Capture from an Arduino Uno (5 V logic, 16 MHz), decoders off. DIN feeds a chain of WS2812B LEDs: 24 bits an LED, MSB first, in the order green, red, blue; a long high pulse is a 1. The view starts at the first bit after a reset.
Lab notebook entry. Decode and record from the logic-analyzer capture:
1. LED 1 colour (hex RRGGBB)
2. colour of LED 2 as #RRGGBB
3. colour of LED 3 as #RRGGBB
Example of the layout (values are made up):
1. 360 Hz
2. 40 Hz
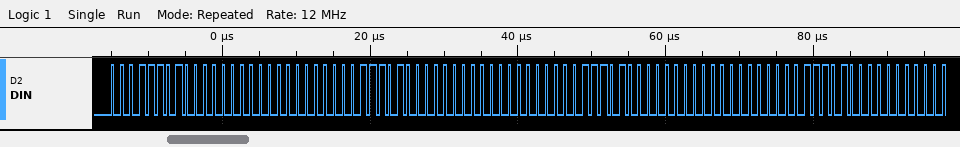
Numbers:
1. #001D00
2. #001D00
3. #001D00
